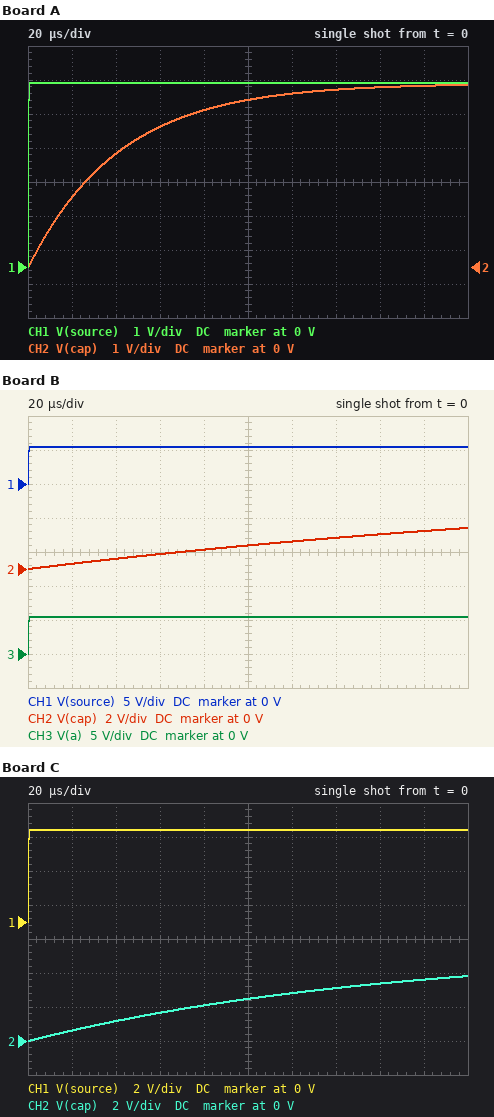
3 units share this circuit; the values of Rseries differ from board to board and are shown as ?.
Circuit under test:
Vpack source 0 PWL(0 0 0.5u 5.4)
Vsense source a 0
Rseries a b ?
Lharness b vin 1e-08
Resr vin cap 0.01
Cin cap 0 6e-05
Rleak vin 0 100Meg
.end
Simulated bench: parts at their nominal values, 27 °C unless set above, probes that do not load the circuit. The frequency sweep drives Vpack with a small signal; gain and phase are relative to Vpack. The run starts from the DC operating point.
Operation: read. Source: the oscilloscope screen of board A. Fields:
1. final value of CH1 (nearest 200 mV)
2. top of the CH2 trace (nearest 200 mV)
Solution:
5.4 V
5.4 V
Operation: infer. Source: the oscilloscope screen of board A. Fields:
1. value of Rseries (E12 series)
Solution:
0.68 Ω
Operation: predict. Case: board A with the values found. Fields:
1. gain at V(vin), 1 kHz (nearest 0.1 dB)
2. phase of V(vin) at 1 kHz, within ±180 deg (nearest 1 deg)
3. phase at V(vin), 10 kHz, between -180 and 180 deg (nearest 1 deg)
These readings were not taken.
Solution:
-0.3 dB
-14 deg
-67 deg
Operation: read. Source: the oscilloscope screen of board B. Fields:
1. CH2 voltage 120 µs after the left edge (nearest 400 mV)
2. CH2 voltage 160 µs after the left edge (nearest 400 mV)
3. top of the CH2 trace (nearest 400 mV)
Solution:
1.6 V
2.0 V
2.4 V
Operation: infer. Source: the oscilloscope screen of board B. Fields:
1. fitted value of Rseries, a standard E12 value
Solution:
5.6 Ω
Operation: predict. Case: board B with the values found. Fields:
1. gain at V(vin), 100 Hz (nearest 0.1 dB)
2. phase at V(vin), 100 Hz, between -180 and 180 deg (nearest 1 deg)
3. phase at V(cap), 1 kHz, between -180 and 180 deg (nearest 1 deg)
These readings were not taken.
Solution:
-0.2 dB
-12 deg
-65 deg
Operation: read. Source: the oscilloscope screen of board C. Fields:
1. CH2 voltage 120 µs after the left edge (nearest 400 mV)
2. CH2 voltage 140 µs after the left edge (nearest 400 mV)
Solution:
2.8 V
3.2 V
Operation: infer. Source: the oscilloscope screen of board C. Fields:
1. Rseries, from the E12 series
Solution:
2.7 Ω
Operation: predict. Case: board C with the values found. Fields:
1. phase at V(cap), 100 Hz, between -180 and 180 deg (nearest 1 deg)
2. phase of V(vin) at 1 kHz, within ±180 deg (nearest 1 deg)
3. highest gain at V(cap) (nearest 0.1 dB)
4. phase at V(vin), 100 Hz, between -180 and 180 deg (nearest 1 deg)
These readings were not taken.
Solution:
-6 deg
-45 deg
0 dB
-6 deg
